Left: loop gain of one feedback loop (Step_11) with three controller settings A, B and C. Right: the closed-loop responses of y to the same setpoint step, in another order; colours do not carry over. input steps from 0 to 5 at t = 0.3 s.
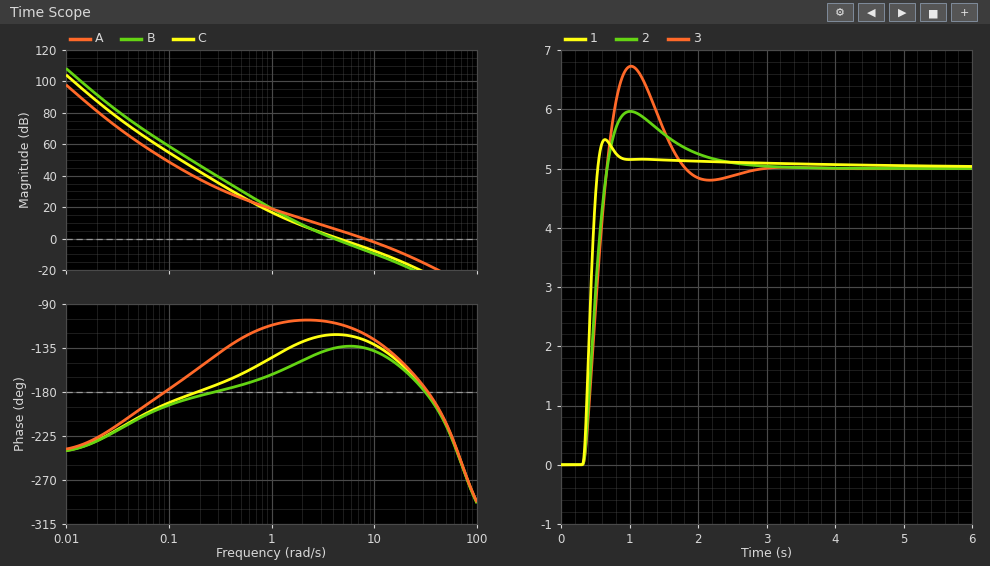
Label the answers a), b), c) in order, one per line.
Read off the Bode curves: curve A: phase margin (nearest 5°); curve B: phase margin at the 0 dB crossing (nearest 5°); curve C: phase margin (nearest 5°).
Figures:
a) 60°
b) 45°
c) 60°
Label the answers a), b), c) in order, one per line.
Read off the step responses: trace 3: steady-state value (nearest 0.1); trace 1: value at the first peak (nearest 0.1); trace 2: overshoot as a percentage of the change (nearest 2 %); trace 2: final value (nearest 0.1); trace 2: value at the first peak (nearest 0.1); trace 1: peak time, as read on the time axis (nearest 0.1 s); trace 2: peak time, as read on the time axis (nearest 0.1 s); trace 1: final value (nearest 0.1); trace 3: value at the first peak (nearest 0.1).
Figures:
a) 5.0
b) 5.5
c) 20 %
d) 5.0
e) 6.0
f) 0.6 s
g) 1.0 s
h) 5.0
i) 6.7
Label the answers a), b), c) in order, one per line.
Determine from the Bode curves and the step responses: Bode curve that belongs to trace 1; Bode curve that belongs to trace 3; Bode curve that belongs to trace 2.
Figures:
a) A
b) B
c) C
